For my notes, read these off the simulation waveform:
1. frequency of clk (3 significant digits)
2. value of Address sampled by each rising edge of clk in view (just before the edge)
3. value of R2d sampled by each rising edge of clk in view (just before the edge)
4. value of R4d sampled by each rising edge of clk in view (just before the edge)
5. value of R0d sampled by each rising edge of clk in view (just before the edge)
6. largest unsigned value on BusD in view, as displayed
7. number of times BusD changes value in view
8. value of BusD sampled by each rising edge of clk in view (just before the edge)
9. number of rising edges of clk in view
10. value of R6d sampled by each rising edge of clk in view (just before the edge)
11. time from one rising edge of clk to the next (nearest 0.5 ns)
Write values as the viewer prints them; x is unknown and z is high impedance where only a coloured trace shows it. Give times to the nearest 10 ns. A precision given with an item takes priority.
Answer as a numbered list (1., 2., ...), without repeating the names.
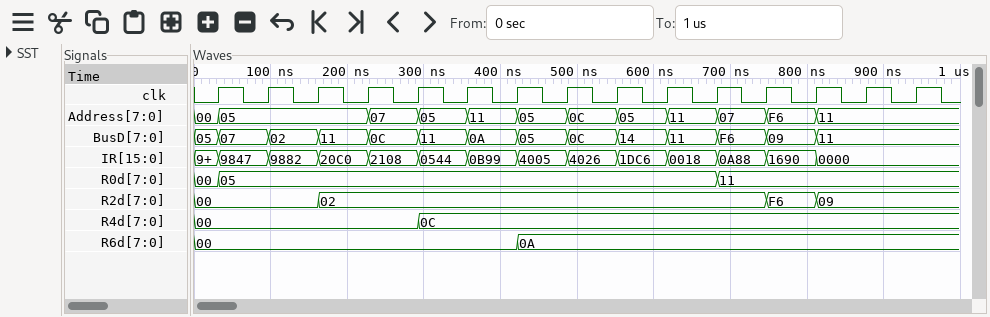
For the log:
1. 15.4 MHz
2. 00, 05, 05, 05, 07, 05, 11, 05, 0C, 05, 11, 07, F6, 11, 11
3. 00, 00, 00, 02, 02, 02, 02, 02, 02, 02, 02, 02, F6, 09, 09
4. 00, 00, 00, 00, 00, 0C, 0C, 0C, 0C, 0C, 0C, 0C, 0C, 0C, 0C
5. 00, 05, 05, 05, 05, 05, 05, 05, 05, 05, 05, 11, 11, 11, 11
6. F6
7. 13
8. 05, 07, 02, 11, 0C, 11, 0A, 05, 0C, 14, 11, F6, 09, 11, 11
9. 15
10. 00, 00, 00, 00, 00, 00, 00, 0A, 0A, 0A, 0A, 0A, 0A, 0A, 0A
11. 65 ns
